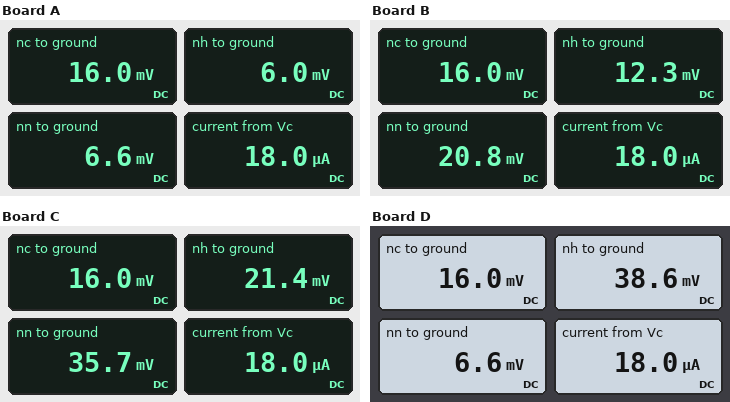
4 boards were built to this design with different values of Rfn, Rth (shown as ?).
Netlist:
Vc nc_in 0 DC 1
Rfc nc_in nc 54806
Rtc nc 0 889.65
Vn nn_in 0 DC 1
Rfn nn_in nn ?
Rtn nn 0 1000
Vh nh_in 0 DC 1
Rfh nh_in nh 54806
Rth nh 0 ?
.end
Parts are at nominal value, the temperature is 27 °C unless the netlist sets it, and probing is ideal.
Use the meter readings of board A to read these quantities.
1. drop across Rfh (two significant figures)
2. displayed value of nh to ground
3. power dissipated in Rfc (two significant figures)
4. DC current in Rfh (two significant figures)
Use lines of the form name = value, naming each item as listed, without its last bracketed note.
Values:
drop across Rfh = 990 mV
displayed value of nh to ground = 6.0 mV
power dissipated in Rfc = 18 µW
DC current in Rfh = 18 µA
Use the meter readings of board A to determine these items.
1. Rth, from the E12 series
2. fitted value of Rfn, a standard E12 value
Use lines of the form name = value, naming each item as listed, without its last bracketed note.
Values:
Rth, from the E12 series = 330 Ω
fitted value of Rfn, a standard E12 value = 150 kΩ
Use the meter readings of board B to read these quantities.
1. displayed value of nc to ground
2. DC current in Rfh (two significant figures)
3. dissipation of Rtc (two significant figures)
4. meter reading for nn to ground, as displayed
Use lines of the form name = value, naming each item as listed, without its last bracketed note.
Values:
displayed value of nc to ground = 16.0 mV
DC current in Rfh = 18 µA
dissipation of Rtc = 290 nW
meter reading for nn to ground, as displayed = 20.8 mV
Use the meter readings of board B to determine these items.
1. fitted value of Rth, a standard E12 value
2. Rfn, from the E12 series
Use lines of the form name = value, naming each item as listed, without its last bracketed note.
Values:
fitted value of Rth, a standard E12 value = 680 Ω
Rfn, from the E12 series = 47 kΩ
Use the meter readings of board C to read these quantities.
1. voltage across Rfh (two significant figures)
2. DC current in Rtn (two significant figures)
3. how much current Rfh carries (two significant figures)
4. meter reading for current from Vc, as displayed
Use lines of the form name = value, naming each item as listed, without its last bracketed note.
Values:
voltage across Rfh = 980 mV
DC current in Rtn = 36 µA
how much current Rfh carries = 18 µA
meter reading for current from Vc, as displayed = 18.0 µA
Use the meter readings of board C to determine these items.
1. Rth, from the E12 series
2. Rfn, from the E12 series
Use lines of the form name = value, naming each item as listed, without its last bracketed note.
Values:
Rth, from the E12 series = 1.2 kΩ
Rfn, from the E12 series = 27 kΩ
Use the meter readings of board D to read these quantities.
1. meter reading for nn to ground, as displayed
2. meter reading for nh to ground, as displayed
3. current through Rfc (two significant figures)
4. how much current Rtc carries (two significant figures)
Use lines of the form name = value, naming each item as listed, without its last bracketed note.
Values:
meter reading for nn to ground, as displayed = 6.6 mV
meter reading for nh to ground, as displayed = 38.6 mV
current through Rfc = 18 µA
how much current Rtc carries = 18 µA
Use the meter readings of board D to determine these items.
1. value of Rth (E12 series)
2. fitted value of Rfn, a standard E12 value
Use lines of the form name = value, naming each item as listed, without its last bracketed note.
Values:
value of Rth = 2.2 kΩ
fitted value of Rfn, a standard E12 value = 150 kΩ
